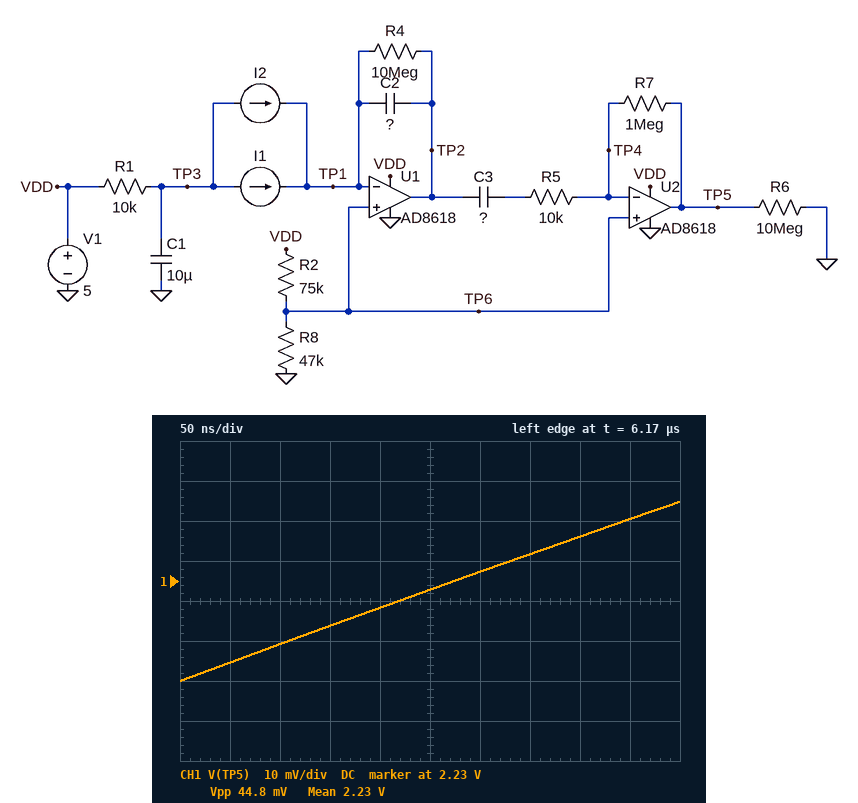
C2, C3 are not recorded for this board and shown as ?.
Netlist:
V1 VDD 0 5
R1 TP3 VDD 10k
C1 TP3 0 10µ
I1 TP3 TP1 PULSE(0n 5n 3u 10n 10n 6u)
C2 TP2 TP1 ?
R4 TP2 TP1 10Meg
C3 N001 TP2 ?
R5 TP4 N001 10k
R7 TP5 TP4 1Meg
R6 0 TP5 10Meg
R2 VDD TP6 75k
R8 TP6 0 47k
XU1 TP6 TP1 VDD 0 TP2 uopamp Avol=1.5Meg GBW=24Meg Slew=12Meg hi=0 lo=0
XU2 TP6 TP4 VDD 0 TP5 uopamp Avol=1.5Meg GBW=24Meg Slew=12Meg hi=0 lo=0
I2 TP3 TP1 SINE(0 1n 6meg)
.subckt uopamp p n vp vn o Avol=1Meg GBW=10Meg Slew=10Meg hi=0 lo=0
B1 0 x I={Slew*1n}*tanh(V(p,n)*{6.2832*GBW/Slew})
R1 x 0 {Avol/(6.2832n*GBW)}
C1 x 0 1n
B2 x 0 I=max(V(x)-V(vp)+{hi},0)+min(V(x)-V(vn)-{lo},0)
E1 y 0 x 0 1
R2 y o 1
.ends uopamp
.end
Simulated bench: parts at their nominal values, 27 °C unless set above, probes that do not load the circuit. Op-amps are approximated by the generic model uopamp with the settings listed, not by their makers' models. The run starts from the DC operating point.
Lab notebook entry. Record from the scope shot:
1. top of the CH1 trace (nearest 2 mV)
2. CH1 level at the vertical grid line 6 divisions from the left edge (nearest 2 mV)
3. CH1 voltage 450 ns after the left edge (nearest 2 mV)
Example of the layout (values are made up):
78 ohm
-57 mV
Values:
2.250 V
2.232 V
2.246 V
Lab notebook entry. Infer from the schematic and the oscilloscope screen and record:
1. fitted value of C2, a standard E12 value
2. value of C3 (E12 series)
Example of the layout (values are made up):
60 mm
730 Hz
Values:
3.9 pF
820 pF
